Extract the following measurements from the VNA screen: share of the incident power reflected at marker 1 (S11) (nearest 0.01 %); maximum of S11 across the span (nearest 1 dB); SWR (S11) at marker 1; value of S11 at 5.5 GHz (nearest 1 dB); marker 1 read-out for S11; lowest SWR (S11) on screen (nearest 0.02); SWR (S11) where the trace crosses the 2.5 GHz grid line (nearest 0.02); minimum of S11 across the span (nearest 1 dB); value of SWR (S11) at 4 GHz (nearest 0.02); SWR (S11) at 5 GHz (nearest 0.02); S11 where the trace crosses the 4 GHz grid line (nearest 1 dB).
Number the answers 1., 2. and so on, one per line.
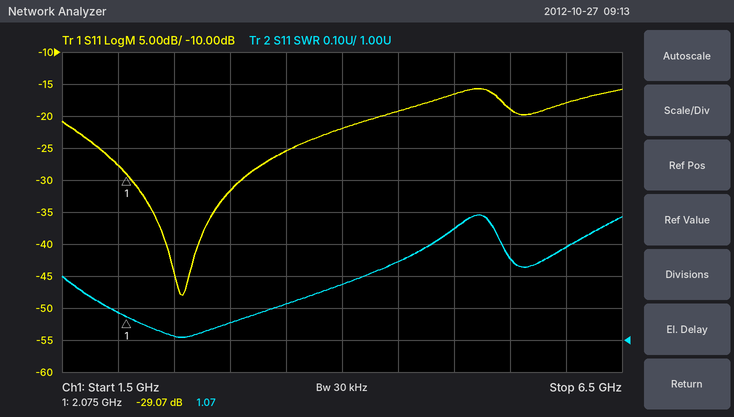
1. 0.12 %
2. -16 dB
3. 1.07
4. -19 dB
5. -29.07 dB
6. 1.00
7. 1.02
8. -48 dB
9. 1.18
10. 1.34
11. -22 dB
